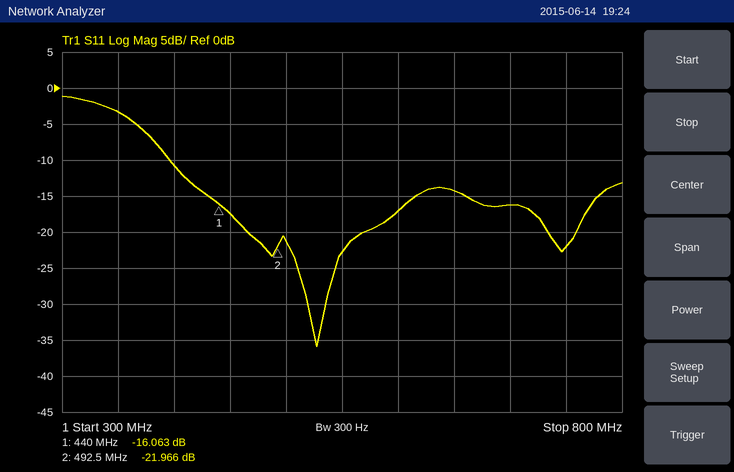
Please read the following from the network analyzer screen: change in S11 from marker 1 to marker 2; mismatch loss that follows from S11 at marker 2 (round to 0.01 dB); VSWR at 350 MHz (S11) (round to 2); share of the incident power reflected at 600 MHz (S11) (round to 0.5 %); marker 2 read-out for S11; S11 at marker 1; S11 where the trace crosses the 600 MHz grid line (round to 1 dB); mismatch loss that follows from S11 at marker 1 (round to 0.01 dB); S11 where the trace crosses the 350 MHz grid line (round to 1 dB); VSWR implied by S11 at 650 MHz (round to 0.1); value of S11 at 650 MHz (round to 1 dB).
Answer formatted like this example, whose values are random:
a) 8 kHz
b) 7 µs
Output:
a) -5.903 dB
b) 0.03 dB
c) 6
d) 2.0 %
e) -21.966 dB
f) -16.063 dB
g) -17 dB
h) 0.11 dB
i) -3 dB
j) 1.5
k) -14 dB
